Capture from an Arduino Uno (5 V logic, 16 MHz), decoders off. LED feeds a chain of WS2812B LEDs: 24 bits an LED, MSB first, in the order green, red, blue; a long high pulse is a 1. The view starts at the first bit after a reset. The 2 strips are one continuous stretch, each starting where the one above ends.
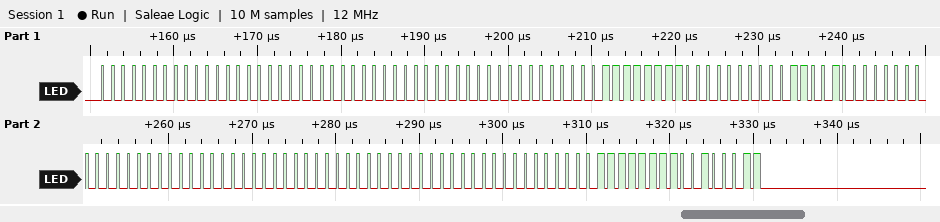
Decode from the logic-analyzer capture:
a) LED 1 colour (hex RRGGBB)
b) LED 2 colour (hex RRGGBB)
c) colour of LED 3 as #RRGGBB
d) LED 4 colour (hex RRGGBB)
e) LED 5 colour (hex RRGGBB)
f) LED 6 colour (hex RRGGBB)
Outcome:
#000000
#000000
#00FF32
#000000
#000000
#FF0023
